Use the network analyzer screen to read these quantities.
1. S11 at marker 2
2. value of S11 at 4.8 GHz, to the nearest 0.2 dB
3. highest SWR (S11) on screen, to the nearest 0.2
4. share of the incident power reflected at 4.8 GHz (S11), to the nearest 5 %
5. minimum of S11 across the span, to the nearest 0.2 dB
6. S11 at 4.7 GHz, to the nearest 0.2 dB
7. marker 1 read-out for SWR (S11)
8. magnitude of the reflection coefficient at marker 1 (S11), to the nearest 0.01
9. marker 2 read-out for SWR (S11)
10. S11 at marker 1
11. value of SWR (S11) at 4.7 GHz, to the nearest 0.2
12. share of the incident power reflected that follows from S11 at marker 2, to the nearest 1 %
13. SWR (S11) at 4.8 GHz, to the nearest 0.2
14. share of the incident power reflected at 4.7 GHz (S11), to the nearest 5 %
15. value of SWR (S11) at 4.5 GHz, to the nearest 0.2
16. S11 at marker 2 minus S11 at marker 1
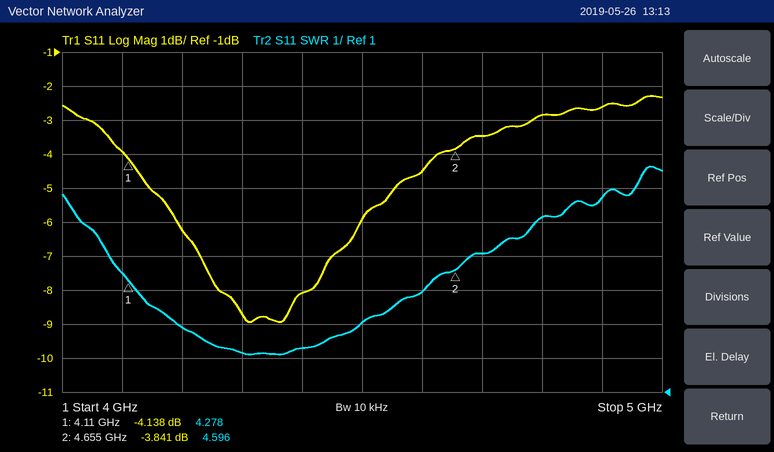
-3.841 dB
-2.8 dB
7.6
50 %
-9.0 dB
-3.4 dB
4.278
0.62
4.596
-4.138 dB
5.0
41 %
6.2
45 %
3.0
0.297 dB
